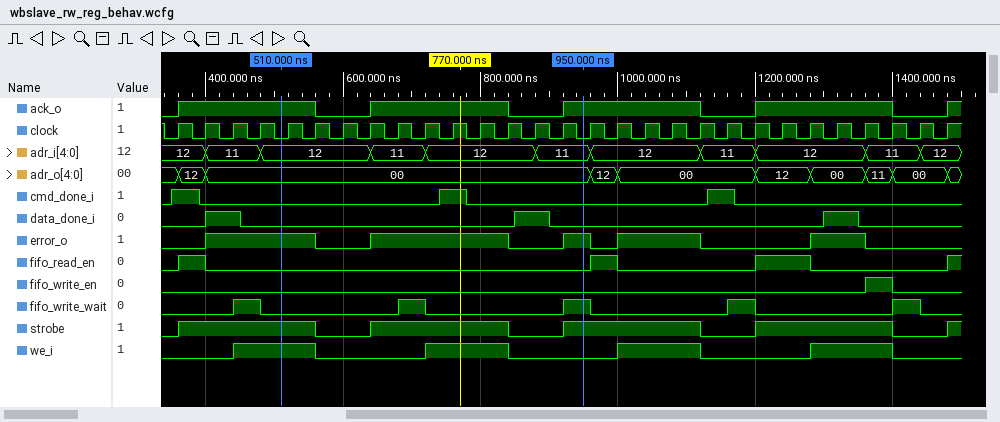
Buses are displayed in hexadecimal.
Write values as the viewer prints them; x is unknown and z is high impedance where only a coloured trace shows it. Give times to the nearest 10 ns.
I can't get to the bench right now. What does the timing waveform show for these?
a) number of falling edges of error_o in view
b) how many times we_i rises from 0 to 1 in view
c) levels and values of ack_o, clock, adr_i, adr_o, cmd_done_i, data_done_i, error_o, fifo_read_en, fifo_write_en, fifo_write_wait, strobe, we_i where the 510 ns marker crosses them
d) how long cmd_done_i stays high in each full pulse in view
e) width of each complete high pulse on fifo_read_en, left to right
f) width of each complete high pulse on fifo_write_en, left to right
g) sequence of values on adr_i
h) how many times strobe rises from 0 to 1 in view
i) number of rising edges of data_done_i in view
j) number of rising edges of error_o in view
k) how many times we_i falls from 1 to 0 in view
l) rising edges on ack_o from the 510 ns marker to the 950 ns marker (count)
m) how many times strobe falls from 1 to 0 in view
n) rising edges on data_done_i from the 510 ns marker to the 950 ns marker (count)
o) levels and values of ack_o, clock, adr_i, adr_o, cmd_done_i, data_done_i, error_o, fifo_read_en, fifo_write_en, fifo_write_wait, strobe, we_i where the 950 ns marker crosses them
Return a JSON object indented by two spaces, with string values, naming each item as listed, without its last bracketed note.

{
  "number of falling edges of error_o in view": "5",
  "how many times we_i rises from 0 to 1 in view": "4",
  "levels and values of ack_o, clock, adr_i, adr_o, cmd_done_i, data_done_i, error_o, fifo_read_en, fifo_write_en, fifo_write_wait, strobe, we_i where the 510 ns marker crosses them": "ack_o=1, clock=0, adr_i=12, adr_o=00, cmd_done_i=0, data_done_i=0, error_o=1, fifo_read_en=0, fifo_write_en=0, fifo_write_wait=0, strobe=1, we_i=1",
  "how long cmd_done_i stays high in each full pulse in view": "40 ns, 40 ns, 40 ns",
  "width of each complete high pulse on fifo_read_en, left to right": "40 ns, 40 ns, 80 ns",
  "width of each complete high pulse on fifo_write_en, left to right": "40 ns",
  "sequence of values on adr_i": "12, 11, 12, 11, 12, 11, 12, 11, 12, 11, 12",
  "how many times strobe rises from 0 to 1 in view": "5",
  "number of rising edges of data_done_i in view": "3",
  "number of rising edges of error_o in view": "5",
  "how many times we_i falls from 1 to 0 in view": "4",
  "rising edges on ack_o from the 510 ns marker to the 950 ns marker": "2",
  "how many times strobe falls from 1 to 0 in view": "4",
  "rising edges on data_done_i from the 510 ns marker to the 950 ns marker": "1",
  "levels and values of ack_o, clock, adr_i, adr_o, cmd_done_i, data_done_i, error_o, fifo_read_en, fifo_write_en, fifo_write_wait, strobe, we_i where the 950 ns marker crosses them": "ack_o=1, clock=0, adr_i=11, adr_o=00, cmd_done_i=0, data_done_i=0, error_o=1, fifo_read_en=0, fifo_write_en=0, fifo_write_wait=1, strobe=1, we_i=0"
}
